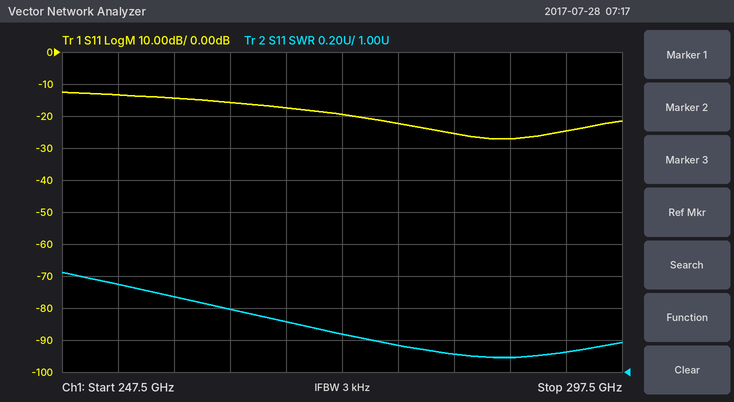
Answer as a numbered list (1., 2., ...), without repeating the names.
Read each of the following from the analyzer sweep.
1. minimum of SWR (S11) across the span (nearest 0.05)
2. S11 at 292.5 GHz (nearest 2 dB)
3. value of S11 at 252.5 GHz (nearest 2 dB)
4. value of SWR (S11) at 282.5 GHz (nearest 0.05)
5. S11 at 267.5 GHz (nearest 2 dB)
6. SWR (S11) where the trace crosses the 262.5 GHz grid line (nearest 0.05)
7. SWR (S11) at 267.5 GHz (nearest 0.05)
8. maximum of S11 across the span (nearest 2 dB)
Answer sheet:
1. 1.10
2. -24 dB
3. -14 dB
4. 1.10
5. -18 dB
6. 1.40
7. 1.30
8. -12 dB
